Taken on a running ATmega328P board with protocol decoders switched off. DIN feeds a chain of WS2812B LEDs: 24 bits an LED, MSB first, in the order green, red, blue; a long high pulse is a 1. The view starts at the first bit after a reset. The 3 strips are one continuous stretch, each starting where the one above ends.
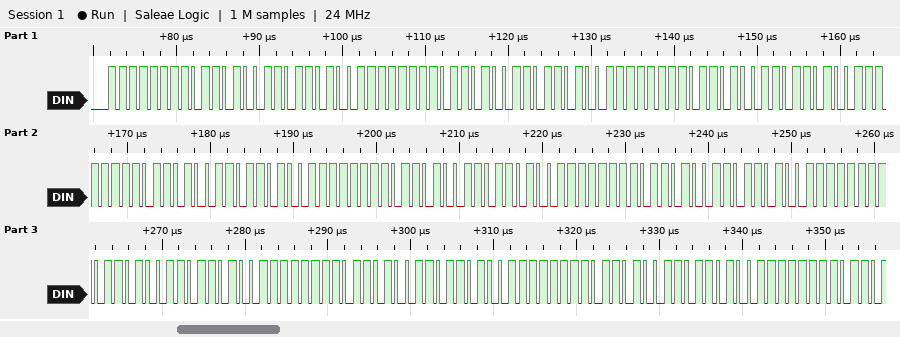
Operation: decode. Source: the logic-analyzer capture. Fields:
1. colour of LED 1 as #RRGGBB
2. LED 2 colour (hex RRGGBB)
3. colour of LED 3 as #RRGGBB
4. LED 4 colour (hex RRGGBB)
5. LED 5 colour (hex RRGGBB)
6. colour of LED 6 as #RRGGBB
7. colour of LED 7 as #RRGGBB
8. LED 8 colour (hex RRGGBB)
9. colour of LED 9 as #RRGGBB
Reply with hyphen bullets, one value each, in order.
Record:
- #69FFB4
- #69FFB4
- #69FFB4
- #69FFB4
- #69FFB4
- #69FFB4
- #69FFB4
- #69FFB4
- #69FFB4
